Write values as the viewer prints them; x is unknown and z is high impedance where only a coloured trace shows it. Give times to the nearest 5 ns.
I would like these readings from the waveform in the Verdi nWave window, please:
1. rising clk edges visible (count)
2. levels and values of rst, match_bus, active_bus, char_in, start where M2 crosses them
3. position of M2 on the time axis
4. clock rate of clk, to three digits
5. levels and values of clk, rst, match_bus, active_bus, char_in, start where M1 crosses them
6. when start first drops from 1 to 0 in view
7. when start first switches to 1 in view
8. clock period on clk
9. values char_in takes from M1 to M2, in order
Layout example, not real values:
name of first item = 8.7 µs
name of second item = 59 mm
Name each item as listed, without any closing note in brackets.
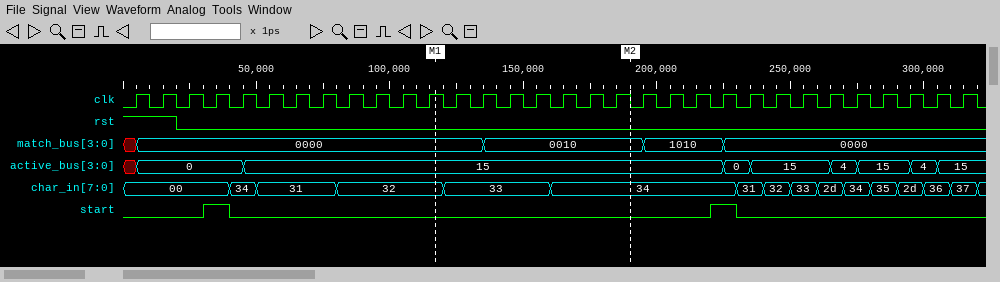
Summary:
rising clk edges visible = 32
levels and values of rst, match_bus, active_bus, char_in, start where M2 crosses them = rst=0, match_bus=0010, active_bus=15, char_in=34, start=0
position of M2 on the time axis = 190 ns
clock rate of clk, to three digits = 100 MHz
levels and values of clk, rst, match_bus, active_bus, char_in, start where M1 crosses them = clk=1, rst=0, match_bus=0000, active_bus=15, char_in=32, start=0
when start first drops from 1 to 0 in view = 40 ns
when start first switches to 1 in view = 30 ns
clock period on clk = 10 ns
values char_in takes from M1 to M2, in order = 32, 33, 34
